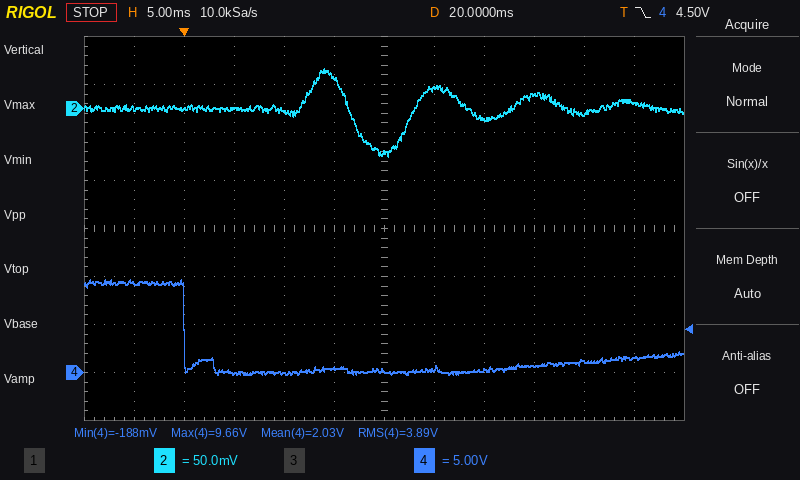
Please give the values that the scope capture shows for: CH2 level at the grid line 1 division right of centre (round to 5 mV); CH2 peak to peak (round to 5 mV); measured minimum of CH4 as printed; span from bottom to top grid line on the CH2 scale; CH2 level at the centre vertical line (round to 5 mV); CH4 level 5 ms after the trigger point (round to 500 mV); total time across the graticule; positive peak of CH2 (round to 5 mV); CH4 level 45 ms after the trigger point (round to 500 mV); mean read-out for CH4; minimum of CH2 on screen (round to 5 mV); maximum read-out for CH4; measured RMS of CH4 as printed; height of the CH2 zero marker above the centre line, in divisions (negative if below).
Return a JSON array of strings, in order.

["20 mV", "90 mV", "-188 mV", "400 mV", "-45 mV", "0.0 V", "60 ms", "40 mV", "1.5 V", "2.03 V", "-50 mV", "9.66 V", "3.89 V", "+2.5 div"]
